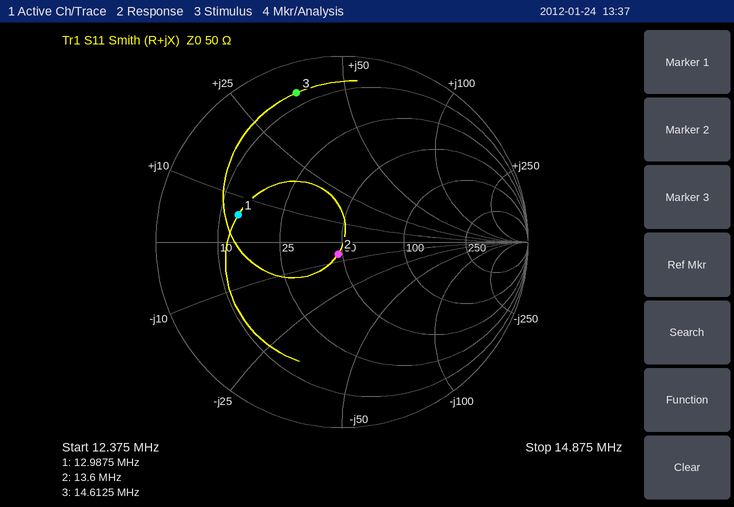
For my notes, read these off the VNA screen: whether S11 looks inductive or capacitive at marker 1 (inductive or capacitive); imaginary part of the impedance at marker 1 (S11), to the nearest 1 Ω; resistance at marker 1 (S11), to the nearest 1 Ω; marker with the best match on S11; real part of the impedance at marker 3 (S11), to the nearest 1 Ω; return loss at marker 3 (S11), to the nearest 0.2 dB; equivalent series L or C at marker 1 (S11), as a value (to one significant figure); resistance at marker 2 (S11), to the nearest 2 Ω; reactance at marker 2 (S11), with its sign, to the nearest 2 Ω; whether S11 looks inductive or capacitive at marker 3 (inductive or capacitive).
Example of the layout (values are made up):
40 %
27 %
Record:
inductive
+6 Ω
14 Ω
marker 2
7 Ω
1.6 dB
70 nH
48 Ω
-6 Ω
inductive
